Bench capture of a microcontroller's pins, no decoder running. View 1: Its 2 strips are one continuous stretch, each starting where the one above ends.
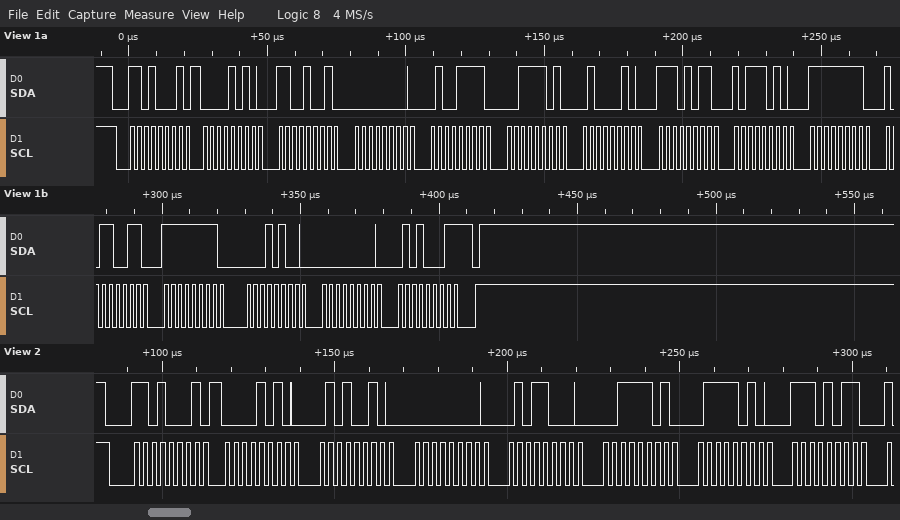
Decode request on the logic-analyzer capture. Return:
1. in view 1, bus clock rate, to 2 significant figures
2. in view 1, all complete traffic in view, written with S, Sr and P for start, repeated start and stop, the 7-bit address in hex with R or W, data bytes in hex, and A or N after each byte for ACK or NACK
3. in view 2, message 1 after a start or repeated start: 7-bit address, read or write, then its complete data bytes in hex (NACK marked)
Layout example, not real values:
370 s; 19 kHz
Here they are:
400 kHz; S 68R A 0A A C9 A 00 A 4F A 3D A 42 A EB A BA A FF A B3 A FF A 14 A 00 A 51 N P; 0x68 read: 0A 52 00 58 3D 7A EB
